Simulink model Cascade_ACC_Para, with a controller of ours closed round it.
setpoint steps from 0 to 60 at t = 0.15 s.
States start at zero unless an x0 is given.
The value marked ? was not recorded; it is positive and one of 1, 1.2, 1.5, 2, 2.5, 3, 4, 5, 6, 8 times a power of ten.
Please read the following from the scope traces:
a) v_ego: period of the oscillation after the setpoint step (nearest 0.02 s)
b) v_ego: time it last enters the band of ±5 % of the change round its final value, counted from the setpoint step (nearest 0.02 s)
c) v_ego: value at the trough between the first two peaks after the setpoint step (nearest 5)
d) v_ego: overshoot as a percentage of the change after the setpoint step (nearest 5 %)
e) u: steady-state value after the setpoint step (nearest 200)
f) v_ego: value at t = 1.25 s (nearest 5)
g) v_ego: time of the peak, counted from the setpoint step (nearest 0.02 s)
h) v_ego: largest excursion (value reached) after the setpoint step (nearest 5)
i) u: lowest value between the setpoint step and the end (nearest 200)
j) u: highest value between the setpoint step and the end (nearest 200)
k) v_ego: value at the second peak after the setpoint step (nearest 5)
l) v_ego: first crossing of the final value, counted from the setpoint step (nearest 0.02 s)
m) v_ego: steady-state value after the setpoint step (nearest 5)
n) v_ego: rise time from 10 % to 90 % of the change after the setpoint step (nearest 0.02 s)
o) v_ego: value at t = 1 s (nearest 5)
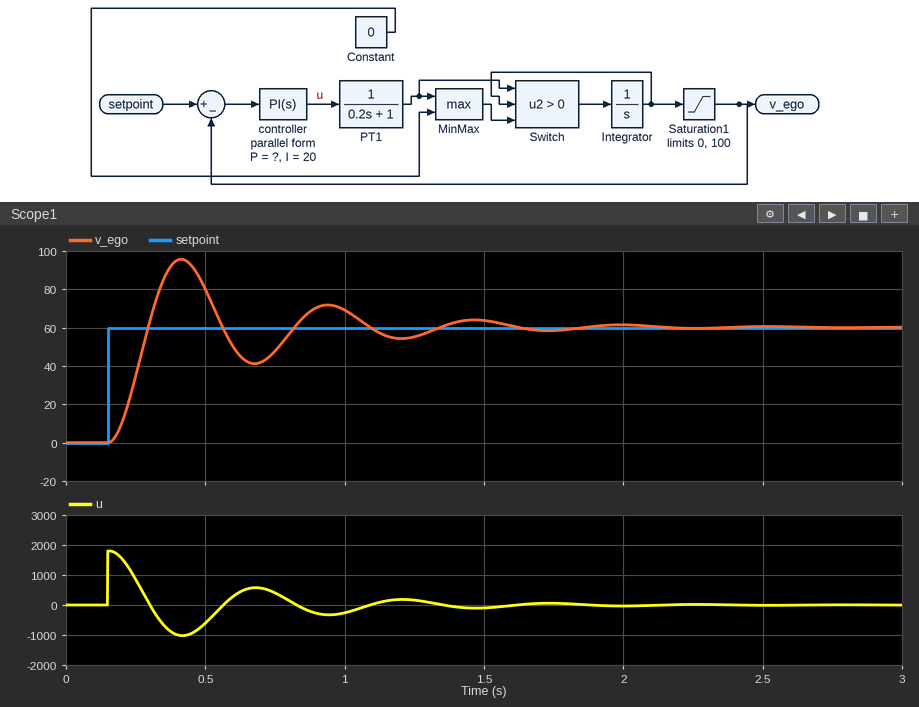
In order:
0.52 s
1.38 s
40
60 %
0
55
0.26 s
95
-1000
1800
70
0.14 s
60
0.10 s
70
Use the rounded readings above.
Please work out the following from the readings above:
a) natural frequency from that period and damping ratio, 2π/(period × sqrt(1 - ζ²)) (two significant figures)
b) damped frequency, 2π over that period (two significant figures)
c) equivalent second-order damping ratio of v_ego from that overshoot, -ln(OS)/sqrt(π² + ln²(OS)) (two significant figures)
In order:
12 rad/s
12 rad/s
0.16
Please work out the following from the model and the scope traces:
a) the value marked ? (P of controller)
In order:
30
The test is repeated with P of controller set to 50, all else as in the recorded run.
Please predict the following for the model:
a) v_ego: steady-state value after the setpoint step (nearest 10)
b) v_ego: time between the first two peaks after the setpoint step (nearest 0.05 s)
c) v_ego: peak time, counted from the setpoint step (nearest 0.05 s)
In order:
60
0.40 s
0.20 s
